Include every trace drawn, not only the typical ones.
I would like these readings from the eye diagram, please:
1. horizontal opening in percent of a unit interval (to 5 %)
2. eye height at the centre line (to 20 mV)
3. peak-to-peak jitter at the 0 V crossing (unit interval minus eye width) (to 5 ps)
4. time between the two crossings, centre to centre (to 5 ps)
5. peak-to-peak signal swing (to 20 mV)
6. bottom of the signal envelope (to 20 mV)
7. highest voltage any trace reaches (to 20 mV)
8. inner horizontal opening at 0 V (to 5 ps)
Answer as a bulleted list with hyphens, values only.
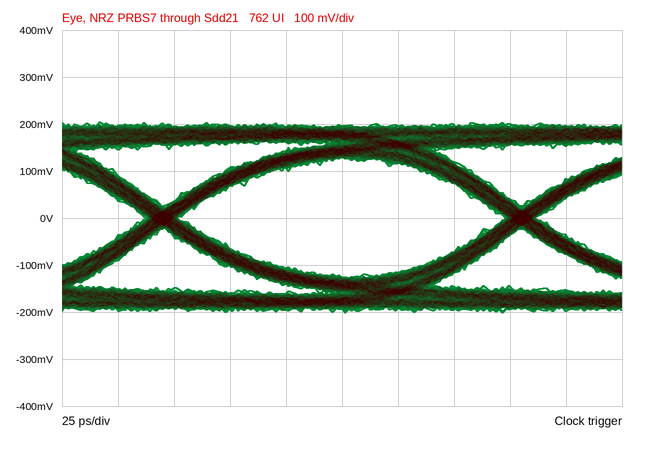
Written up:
- 90 %
- 260 mV
- 15 ps
- 160 ps
- 400 mV
- -200 mV
- 200 mV
- 145 ps
